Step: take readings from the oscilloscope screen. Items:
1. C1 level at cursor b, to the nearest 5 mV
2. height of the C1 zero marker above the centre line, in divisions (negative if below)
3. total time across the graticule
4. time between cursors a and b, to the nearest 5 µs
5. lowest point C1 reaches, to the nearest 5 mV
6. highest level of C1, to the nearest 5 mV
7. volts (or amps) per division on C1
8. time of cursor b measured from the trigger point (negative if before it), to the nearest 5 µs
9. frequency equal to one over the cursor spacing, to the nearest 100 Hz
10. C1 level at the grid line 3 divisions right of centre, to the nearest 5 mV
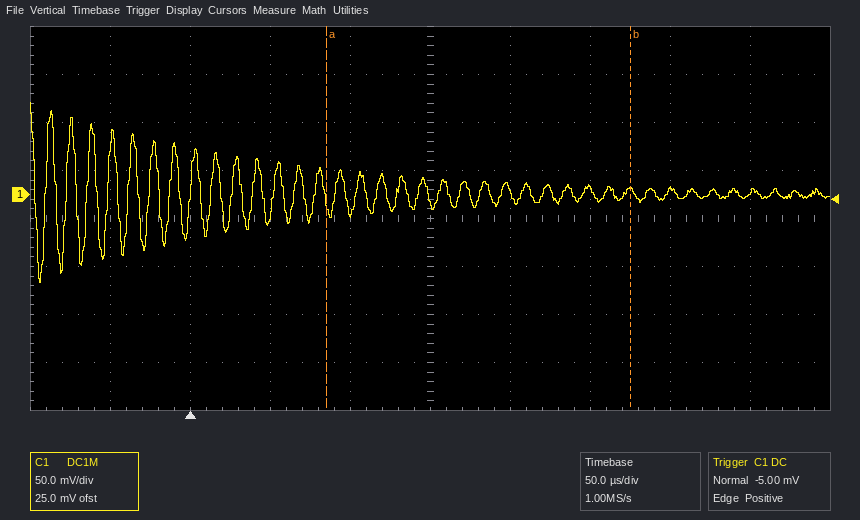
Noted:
5 mV
+0.5 div
500 µs
190 µs
-90 mV
95 mV
50 mV
+275 µs
5.3 kHz
5 mV
